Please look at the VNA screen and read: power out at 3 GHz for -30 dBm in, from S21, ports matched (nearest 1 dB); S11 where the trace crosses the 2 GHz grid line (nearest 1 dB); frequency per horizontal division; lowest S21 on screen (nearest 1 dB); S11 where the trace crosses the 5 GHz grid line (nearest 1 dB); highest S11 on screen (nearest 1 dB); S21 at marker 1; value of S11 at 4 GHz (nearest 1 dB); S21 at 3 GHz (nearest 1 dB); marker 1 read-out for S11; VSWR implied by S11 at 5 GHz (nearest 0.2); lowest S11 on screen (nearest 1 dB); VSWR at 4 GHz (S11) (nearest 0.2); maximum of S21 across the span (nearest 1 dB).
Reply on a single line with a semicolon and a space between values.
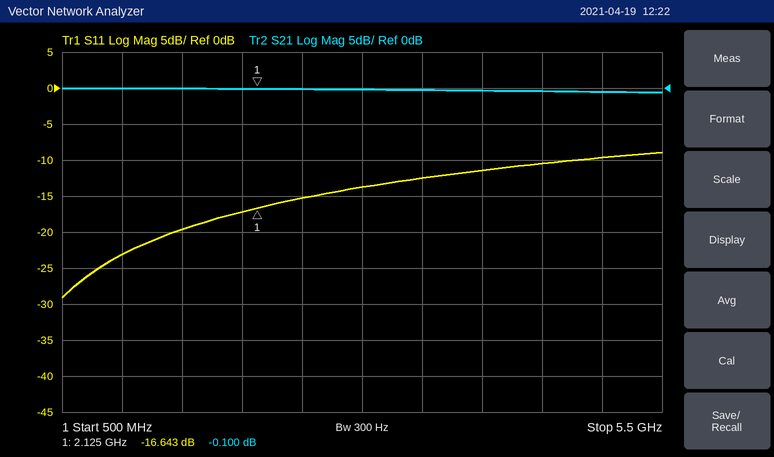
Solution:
-30 dBm; -17 dB; 500 MHz; -1 dB; -10 dB; -9 dB; -0.100 dB; -11 dB; 0 dB; -16.643 dB; 2.0; -29 dB; 1.8; 0 dB
